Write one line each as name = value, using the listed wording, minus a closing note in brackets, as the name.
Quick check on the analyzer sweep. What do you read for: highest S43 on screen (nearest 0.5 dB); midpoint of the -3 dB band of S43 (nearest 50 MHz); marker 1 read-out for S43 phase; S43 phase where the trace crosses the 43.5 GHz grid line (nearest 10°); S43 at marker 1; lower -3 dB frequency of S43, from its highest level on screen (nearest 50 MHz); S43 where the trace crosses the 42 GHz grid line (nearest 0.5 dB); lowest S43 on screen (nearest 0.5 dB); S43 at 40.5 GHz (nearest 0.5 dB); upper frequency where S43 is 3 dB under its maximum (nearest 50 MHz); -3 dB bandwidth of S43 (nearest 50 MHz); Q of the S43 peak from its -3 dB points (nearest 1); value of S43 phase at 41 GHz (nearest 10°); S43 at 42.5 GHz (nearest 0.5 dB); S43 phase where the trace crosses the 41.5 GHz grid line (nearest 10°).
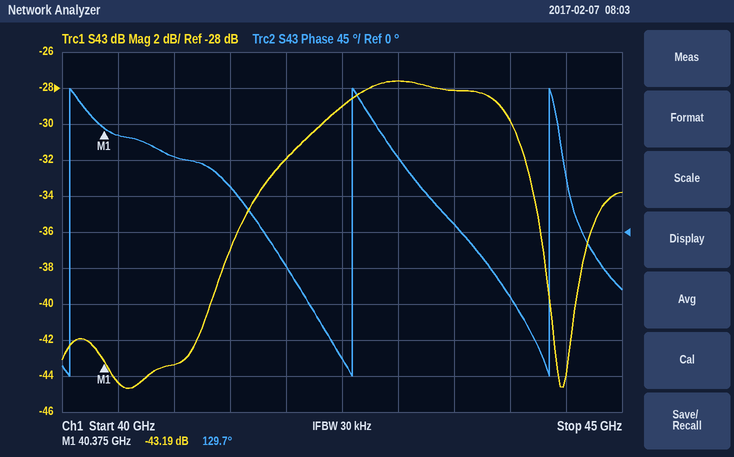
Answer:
highest S43 on screen = -27.5 dB
midpoint of the -3 dB band of S43 = 43.15 GHz
marker 1 read-out for S43 phase = 129.7°
S43 phase where the trace crosses the 43.5 GHz grid line = 10°
S43 at marker 1 = -43.19 dB
lower -3 dB frequency of S43, from its highest level on screen = 42.20 GHz
S43 where the trace crosses the 42 GHz grid line = -32.0 dB
lowest S43 on screen = -44.5 dB
S43 at 40.5 GHz = -44.5 dB
upper frequency where S43 is 3 dB under its maximum = 44.05 GHz
-3 dB bandwidth of S43 = 1.85 GHz
Q of the S43 peak from its -3 dB points = 23
value of S43 phase at 41 GHz = 90°
S43 at 42.5 GHz = -29.0 dB
S43 phase where the trace crosses the 41.5 GHz grid line = 60°
